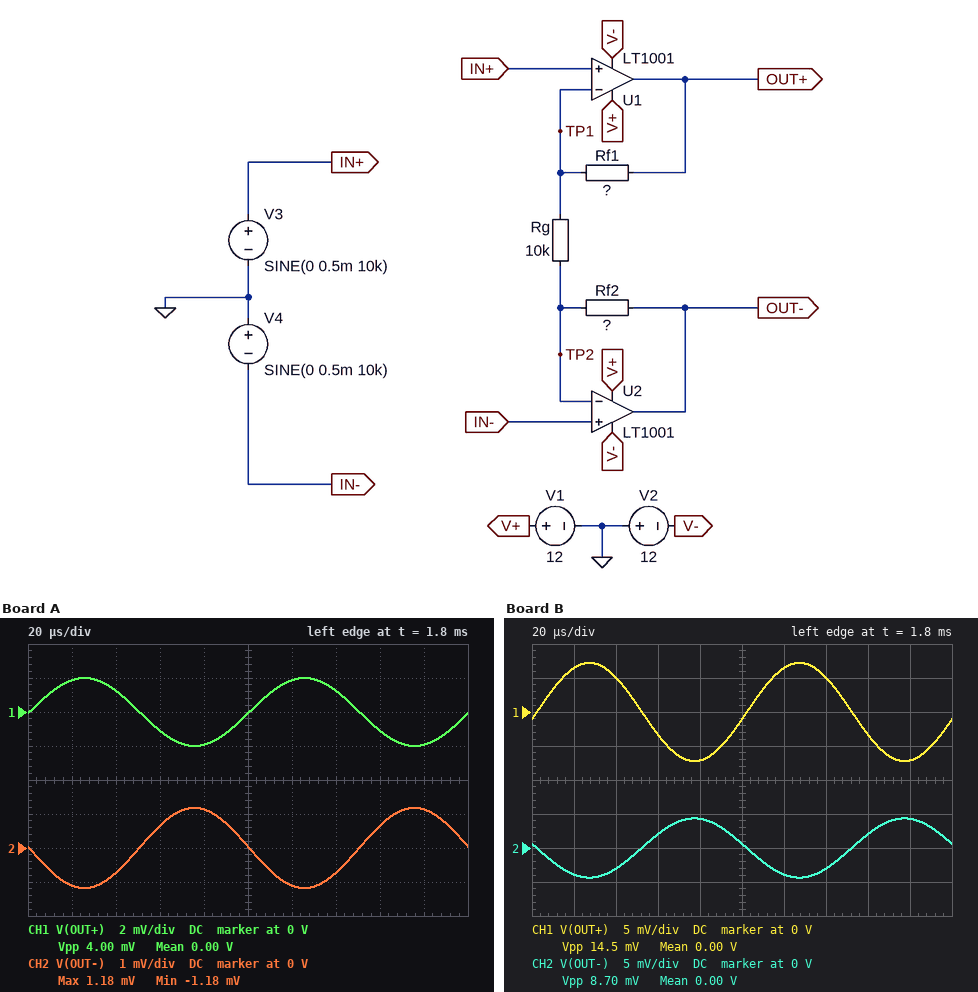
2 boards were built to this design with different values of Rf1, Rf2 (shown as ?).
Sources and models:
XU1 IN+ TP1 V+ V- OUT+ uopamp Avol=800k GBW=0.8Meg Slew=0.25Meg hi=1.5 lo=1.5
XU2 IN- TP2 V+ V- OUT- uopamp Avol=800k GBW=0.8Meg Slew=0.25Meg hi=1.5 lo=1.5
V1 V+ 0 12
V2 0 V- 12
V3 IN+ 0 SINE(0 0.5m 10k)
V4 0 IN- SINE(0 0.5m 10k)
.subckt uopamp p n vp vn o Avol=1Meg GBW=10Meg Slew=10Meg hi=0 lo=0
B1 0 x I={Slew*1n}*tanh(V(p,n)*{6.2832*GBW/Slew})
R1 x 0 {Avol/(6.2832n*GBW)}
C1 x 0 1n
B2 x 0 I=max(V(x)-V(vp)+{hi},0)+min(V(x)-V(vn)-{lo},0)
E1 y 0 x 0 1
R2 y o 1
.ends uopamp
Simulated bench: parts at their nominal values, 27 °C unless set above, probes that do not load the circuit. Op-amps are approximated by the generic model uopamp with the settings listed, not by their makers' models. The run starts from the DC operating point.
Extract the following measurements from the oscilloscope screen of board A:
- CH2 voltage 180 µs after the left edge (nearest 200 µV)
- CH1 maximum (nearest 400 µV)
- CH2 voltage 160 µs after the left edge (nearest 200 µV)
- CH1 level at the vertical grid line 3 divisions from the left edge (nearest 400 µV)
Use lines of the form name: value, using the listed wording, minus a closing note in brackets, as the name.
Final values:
CH2 voltage 180 µs after the left edge: 1.2 mV
CH1 maximum: 2.0 mV
CH2 voltage 160 µs after the left edge: 600 µV
CH1 level at the vertical grid line 3 divisions from the left edge: -1.2 mV
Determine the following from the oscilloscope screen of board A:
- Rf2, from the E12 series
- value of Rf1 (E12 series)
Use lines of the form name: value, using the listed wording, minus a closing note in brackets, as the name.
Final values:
Rf2, from the E12 series: 6.8 kΩ
value of Rf1: 15 kΩ
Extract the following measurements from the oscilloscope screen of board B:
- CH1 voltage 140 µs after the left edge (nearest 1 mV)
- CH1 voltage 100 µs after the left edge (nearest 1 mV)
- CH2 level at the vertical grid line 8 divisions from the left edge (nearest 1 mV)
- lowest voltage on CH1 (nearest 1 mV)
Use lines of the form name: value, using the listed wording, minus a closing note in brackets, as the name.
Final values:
CH1 voltage 140 µs after the left edge: 5 mV
CH1 voltage 100 µs after the left edge: -1 mV
CH2 level at the vertical grid line 8 divisions from the left edge: 2 mV
lowest voltage on CH1: -7 mV
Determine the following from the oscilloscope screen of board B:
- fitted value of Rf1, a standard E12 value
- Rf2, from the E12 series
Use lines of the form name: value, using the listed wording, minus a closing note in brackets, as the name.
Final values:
fitted value of Rf1, a standard E12 value: 68 kΩ
Rf2, from the E12 series: 39 kΩ
